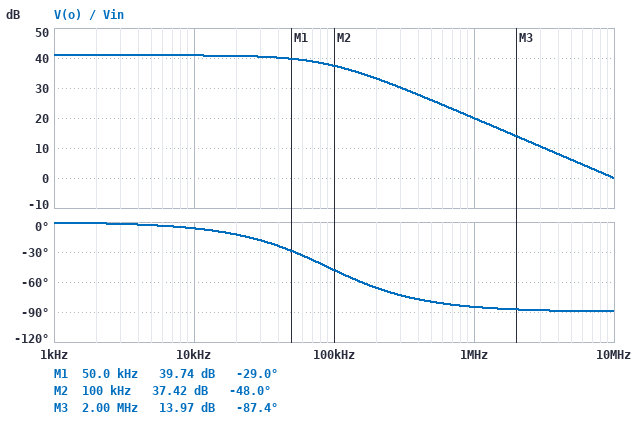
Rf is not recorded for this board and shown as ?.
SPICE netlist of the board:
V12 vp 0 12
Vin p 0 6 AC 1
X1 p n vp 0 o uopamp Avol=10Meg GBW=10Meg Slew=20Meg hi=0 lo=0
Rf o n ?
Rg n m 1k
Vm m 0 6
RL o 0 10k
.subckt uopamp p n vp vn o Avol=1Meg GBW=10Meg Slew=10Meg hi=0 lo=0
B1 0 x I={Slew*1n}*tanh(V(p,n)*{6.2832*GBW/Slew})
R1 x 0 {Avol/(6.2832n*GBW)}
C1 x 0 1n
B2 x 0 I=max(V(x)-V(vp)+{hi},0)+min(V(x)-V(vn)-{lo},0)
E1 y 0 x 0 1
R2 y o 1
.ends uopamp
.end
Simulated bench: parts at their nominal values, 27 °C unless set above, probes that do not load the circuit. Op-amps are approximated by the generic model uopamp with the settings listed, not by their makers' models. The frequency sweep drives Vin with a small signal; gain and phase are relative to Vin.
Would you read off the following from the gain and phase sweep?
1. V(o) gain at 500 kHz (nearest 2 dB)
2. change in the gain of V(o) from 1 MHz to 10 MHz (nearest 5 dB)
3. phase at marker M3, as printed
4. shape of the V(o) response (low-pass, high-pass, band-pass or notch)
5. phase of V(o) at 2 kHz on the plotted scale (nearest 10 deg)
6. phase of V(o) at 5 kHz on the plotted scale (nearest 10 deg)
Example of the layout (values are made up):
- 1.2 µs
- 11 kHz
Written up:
- 26 dB
- -20 dB
- -87.4 deg
- low-pass
- 0 deg
- 0 deg
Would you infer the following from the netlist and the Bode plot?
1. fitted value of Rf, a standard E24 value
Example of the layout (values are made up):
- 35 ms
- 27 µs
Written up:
- 110 kΩ
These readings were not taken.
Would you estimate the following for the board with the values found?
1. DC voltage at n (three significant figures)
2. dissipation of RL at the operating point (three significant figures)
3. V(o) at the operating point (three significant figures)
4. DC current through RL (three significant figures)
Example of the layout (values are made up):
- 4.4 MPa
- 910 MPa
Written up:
- 6.00 V
- 3.60 mW
- 6.00 V
- 600 µA
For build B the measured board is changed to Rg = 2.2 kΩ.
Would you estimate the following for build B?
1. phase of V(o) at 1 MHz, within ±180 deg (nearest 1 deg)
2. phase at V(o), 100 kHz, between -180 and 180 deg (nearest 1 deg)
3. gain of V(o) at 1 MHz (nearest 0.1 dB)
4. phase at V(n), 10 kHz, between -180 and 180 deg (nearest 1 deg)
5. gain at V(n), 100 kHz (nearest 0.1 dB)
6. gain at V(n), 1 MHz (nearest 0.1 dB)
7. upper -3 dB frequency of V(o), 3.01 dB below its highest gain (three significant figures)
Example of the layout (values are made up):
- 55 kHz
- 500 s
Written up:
- -79 deg
- -27 deg
- 19.8 dB
- -3 deg
- -1.0 dB
- -14.3 dB
- 196 kHz
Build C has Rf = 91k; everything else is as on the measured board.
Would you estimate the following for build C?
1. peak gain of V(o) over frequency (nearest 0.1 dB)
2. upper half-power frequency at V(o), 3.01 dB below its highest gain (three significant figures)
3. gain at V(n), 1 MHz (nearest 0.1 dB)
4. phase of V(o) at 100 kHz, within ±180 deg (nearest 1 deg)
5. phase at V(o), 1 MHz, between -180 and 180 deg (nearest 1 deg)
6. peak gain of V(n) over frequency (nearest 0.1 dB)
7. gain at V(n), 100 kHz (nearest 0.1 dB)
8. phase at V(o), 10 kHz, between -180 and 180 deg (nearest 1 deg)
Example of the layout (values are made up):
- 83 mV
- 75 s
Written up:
- 39.3 dB
- 109 kHz
- -19.3 dB
- -43 deg
- -84 deg
- 0 dB
- -2.7 dB
- -5 deg
